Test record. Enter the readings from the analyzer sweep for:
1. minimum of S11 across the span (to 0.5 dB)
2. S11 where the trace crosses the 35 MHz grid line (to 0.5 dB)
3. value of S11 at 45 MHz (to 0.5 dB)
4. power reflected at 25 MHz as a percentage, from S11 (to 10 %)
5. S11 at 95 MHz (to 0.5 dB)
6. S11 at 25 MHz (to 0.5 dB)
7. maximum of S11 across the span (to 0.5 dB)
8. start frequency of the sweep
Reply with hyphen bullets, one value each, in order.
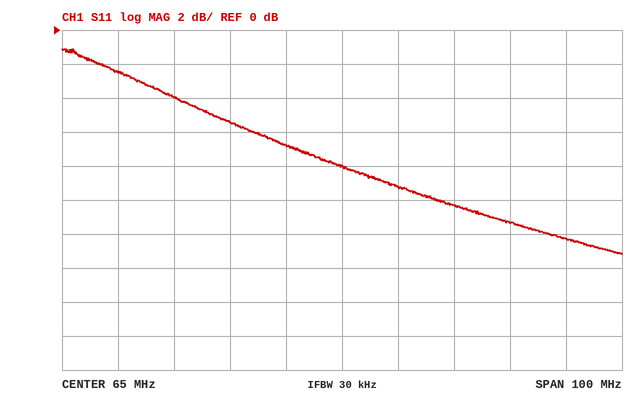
- -13.0 dB
- -4.0 dB
- -5.5 dB
- 60 %
- -11.5 dB
- -2.5 dB
- -1.0 dB
- 15 MHz
